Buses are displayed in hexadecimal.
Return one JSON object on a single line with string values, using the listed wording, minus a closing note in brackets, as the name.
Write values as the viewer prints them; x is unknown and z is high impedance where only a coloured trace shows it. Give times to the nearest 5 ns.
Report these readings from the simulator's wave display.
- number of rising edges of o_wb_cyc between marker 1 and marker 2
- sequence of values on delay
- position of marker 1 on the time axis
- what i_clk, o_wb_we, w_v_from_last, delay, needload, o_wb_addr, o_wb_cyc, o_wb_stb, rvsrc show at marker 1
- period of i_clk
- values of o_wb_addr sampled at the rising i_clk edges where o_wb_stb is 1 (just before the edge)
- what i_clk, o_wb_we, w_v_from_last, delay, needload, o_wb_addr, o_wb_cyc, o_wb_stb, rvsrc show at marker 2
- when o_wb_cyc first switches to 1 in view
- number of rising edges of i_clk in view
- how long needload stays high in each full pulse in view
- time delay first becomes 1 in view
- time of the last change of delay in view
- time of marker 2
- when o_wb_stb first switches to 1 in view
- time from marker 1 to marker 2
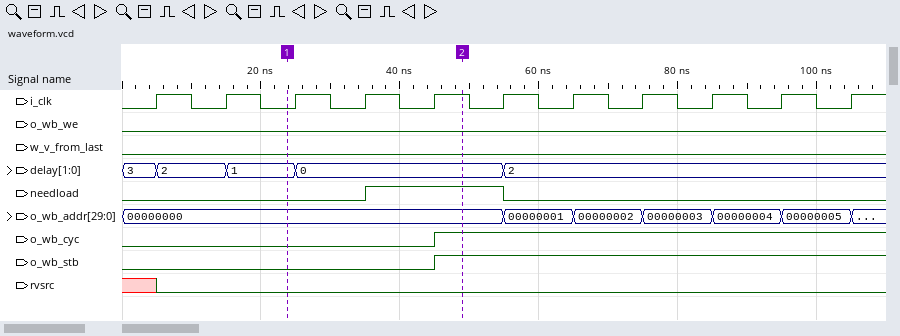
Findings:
{"number of rising edges of o_wb_cyc between marker 1 and marker 2": "1", "sequence of values on delay": "3, 2, 1, 0, 2", "position of marker 1 on the time axis": "25 ns", "what i_clk, o_wb_we, w_v_from_last, delay, needload, o_wb_addr, o_wb_cyc, o_wb_stb, rvsrc show at marker 1": "i_clk=0, o_wb_we=0, w_v_from_last=0, delay=1, needload=0, o_wb_addr=00000000, o_wb_cyc=0, o_wb_stb=0, rvsrc=0", "period of i_clk": "10 ns", "values of o_wb_addr sampled at the rising i_clk edges where o_wb_stb is 1": "00000000, 00000001, 00000002, 00000003, 00000004, 00000005", "what i_clk, o_wb_we, w_v_from_last, delay, needload, o_wb_addr, o_wb_cyc, o_wb_stb, rvsrc show at marker 2": "i_clk=1, o_wb_we=0, w_v_from_last=0, delay=0, needload=1, o_wb_addr=00000000, o_wb_cyc=1, o_wb_stb=1, rvsrc=0", "when o_wb_cyc first switches to 1 in view": "45 ns", "number of rising edges of i_clk in view": "11", "how long needload stays high in each full pulse in view": "20 ns", "time delay first becomes 1 in view": "15 ns", "time of the last change of delay in view": "55 ns", "time of marker 2": "50 ns", "when o_wb_stb first switches to 1 in view": "45 ns", "time from marker 1 to marker 2": "25 ns"}
